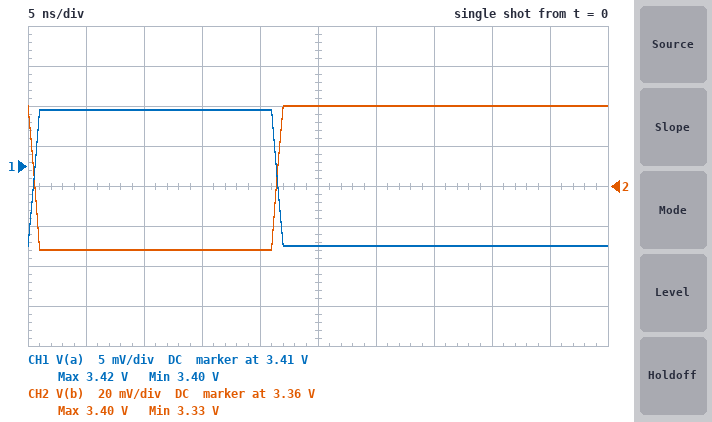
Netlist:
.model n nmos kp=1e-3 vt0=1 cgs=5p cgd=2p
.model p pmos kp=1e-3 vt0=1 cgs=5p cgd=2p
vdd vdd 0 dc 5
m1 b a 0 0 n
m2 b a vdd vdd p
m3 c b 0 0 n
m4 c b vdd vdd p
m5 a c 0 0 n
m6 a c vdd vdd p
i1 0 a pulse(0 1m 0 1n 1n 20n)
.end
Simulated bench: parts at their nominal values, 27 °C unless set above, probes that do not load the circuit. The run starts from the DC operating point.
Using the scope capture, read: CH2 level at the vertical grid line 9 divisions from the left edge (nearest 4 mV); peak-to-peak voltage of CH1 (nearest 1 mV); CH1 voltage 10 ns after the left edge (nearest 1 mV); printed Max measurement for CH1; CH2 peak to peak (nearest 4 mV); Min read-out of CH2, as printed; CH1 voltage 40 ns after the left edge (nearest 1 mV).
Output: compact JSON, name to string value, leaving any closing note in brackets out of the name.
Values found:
{"CH2 level at the vertical grid line 9 divisions from the left edge": "3.400 V", "peak-to-peak voltage of CH1": "17 mV", "CH1 voltage 10 ns after the left edge": "3.417 V", "printed Max measurement for CH1": "3.42 V", "CH2 peak to peak": "72 mV", "Min read-out of CH2, as printed": "3.33 V", "CH1 voltage 40 ns after the left edge": "3.400 V"}
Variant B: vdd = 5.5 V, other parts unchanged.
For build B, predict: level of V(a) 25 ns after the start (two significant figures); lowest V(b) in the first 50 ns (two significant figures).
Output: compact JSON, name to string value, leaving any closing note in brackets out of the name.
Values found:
{"level of V(a) 25 ns after the start": "3.7 V", "lowest V(b) in the first 50 ns": "3.6 V"}
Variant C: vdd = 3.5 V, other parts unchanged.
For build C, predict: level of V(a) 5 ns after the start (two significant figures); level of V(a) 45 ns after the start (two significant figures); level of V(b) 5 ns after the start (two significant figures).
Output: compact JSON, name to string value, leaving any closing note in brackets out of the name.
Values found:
{"level of V(a) 5 ns after the start": "2.7 V", "level of V(a) 45 ns after the start": "2.6 V", "level of V(b) 5 ns after the start": "2.4 V"}
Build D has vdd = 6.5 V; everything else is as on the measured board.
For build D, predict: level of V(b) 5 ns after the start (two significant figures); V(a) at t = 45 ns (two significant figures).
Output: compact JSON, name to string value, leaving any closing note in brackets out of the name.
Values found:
{"level of V(b) 5 ns after the start": "4.1 V", "V(a) at t = 45 ns": "4.2 V"}
